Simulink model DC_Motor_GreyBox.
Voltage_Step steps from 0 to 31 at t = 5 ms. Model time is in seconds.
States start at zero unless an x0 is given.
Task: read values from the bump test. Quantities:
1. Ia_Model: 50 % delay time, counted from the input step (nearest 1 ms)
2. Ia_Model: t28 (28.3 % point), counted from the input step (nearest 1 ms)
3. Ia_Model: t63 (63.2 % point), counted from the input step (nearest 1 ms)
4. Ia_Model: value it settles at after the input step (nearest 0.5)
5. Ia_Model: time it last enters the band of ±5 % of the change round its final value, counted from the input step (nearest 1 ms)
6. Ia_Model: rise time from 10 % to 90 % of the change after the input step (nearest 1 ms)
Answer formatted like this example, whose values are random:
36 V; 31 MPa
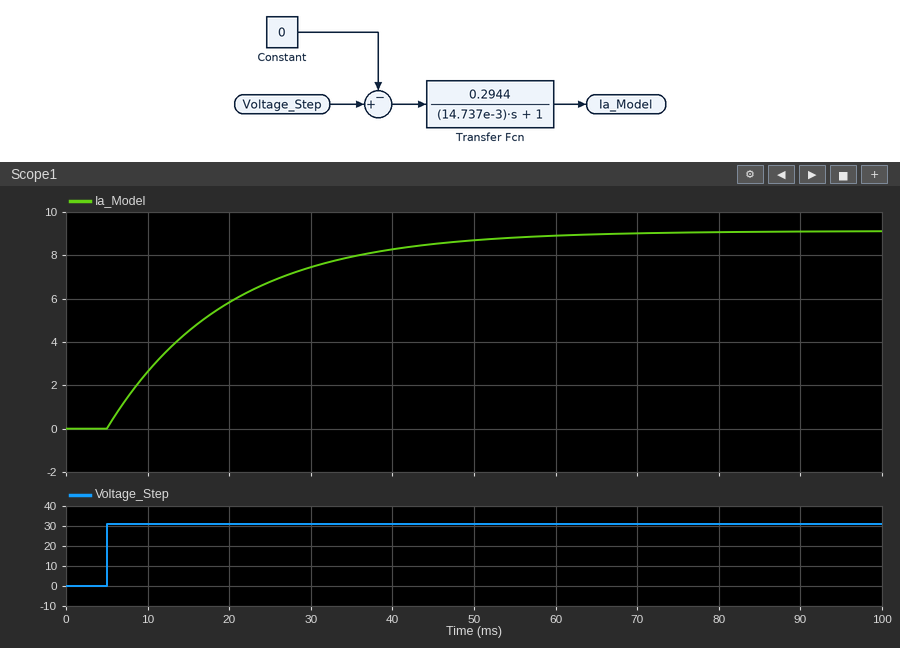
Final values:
10 ms; 5 ms; 15 ms; 9.0; 44 ms; 32 ms
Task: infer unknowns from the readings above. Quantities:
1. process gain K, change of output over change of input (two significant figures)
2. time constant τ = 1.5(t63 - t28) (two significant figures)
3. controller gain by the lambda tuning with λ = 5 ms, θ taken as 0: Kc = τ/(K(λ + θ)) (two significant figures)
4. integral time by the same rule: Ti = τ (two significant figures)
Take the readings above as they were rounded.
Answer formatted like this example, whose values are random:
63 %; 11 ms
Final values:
0.29; 15 ms; 10; 15 ms
